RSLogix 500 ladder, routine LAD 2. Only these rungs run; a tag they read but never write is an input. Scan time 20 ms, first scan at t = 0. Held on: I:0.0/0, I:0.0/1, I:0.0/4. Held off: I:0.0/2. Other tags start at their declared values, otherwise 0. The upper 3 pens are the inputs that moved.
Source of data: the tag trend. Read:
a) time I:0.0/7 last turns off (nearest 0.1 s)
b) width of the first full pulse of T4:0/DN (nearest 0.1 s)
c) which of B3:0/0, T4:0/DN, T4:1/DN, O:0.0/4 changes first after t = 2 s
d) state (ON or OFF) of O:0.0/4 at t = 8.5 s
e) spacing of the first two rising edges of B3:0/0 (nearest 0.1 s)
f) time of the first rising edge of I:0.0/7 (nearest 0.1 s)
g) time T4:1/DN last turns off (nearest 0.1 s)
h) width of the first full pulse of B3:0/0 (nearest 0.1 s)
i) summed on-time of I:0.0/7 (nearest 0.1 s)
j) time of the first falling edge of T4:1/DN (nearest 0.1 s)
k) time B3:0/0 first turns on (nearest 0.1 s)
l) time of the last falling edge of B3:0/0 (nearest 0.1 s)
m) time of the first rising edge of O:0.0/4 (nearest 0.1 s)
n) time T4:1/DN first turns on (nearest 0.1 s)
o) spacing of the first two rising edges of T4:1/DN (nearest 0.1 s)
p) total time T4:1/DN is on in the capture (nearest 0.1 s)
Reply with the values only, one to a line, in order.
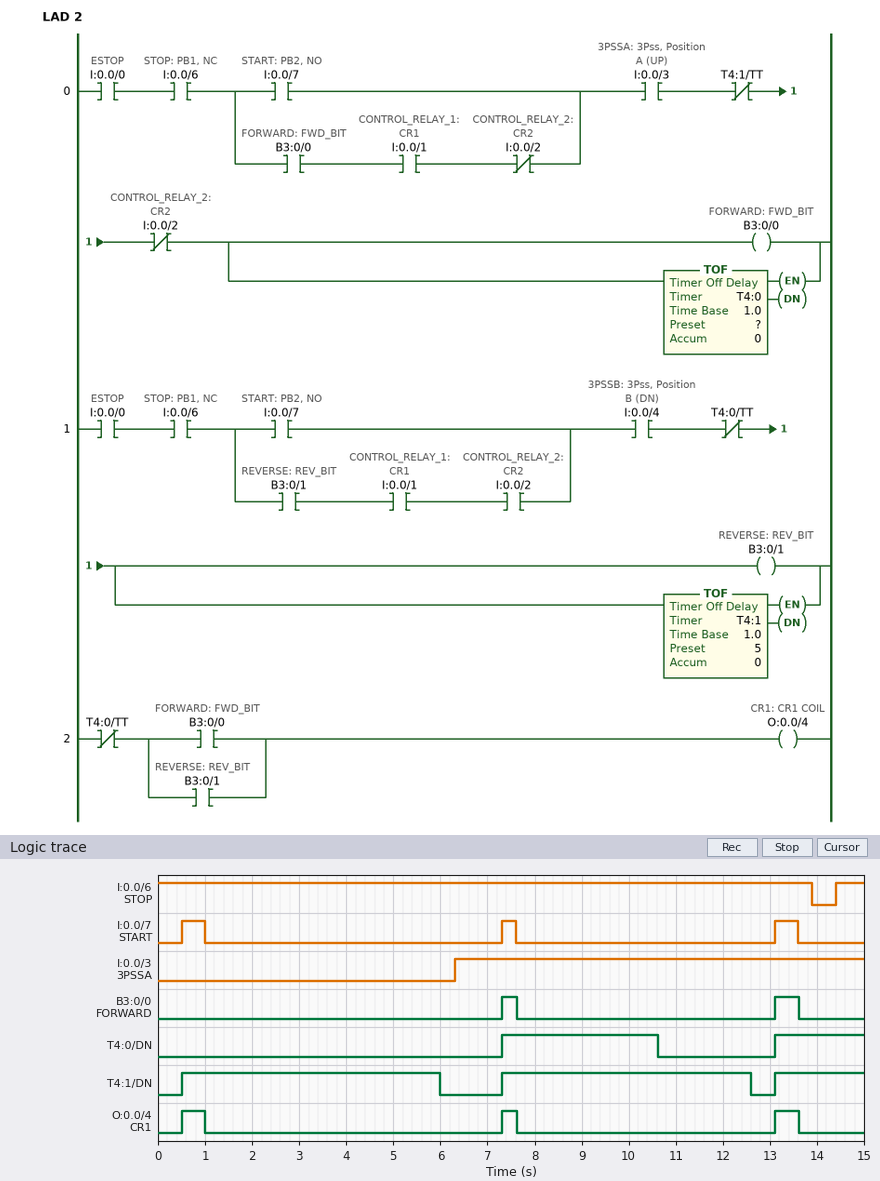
13.6 s
3.3 s
T4:1/DN
OFF
5.8 s
0.5 s
12.6 s
0.3 s
1.3 s
6.0 s
7.3 s
13.6 s
0.5 s
0.5 s
6.8 s
12.7 s
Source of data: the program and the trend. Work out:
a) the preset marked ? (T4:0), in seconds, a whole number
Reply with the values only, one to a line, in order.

3 s
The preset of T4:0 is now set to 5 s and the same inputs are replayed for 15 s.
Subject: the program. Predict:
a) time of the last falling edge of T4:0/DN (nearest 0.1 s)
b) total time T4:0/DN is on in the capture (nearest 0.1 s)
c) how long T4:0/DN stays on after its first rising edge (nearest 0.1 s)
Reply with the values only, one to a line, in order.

12.6 s
7.2 s
5.3 s
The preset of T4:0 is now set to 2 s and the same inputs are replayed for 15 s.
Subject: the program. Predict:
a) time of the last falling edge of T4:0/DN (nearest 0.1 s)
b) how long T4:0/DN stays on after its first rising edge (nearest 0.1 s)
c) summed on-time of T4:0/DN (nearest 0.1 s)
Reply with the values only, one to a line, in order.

9.6 s
2.3 s
4.2 s
